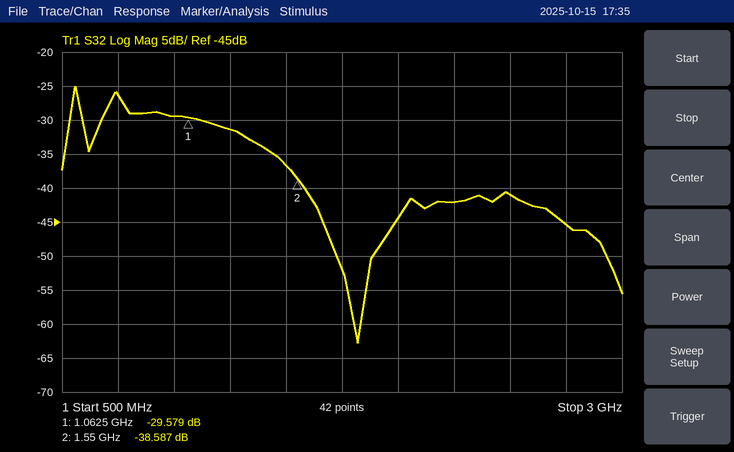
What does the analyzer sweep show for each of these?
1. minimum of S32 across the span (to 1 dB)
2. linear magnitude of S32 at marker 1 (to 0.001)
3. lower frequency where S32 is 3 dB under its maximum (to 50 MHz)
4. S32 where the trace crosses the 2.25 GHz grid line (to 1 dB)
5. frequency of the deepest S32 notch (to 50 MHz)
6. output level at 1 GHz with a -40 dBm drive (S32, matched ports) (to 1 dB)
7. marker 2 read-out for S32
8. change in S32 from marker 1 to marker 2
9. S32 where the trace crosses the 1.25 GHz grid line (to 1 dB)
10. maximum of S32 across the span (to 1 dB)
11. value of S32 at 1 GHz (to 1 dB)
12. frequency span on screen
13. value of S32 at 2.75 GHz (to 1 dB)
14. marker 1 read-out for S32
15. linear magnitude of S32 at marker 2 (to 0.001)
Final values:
-63 dB
0.033
550 MHz
-42 dB
1.80 GHz
-69 dBm
-38.587 dB
-9.008 dB
-31 dB
-25 dB
-29 dB
2.5 GHz
-45 dB
-29.579 dB
0.012
